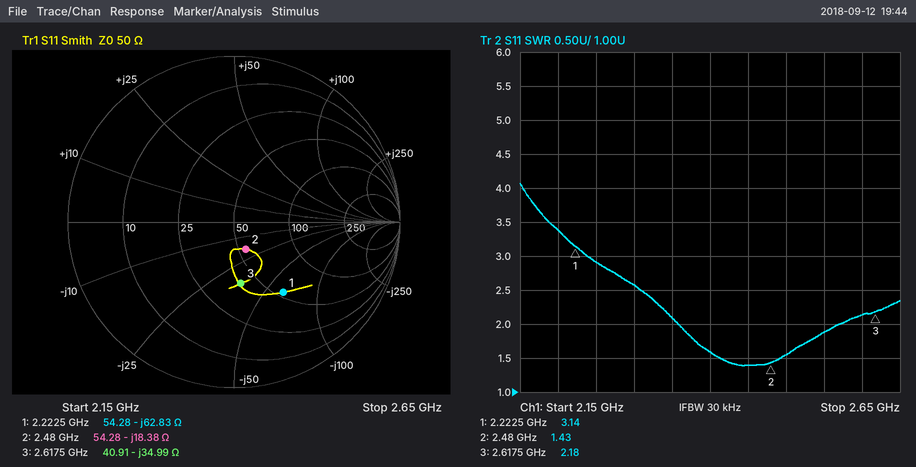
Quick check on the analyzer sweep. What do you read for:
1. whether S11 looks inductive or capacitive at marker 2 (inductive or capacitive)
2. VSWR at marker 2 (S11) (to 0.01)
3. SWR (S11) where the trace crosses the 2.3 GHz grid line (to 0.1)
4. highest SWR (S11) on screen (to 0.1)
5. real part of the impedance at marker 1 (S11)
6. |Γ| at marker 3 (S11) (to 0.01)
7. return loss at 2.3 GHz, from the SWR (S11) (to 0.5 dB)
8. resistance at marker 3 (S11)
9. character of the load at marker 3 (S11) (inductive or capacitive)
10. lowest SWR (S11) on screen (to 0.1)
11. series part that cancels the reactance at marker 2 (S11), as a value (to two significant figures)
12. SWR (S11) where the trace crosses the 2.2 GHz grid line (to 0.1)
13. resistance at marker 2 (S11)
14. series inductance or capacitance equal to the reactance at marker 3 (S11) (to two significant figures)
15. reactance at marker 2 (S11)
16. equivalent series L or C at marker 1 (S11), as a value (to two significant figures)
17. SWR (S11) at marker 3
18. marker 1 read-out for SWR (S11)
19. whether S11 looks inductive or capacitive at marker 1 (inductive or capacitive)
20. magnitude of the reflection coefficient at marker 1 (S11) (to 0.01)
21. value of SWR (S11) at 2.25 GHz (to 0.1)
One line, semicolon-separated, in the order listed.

capacitive; 1.43; 2.6; 4.1; 54.28 Ω; 0.37; 7.0 dB; 40.91 Ω; capacitive; 1.4; 1.2 nH; 3.4; 54.28 Ω; 1.7 pF; -18.38 Ω; 1.1 pF; 2.18; 3.14; capacitive; 0.52; 2.9
